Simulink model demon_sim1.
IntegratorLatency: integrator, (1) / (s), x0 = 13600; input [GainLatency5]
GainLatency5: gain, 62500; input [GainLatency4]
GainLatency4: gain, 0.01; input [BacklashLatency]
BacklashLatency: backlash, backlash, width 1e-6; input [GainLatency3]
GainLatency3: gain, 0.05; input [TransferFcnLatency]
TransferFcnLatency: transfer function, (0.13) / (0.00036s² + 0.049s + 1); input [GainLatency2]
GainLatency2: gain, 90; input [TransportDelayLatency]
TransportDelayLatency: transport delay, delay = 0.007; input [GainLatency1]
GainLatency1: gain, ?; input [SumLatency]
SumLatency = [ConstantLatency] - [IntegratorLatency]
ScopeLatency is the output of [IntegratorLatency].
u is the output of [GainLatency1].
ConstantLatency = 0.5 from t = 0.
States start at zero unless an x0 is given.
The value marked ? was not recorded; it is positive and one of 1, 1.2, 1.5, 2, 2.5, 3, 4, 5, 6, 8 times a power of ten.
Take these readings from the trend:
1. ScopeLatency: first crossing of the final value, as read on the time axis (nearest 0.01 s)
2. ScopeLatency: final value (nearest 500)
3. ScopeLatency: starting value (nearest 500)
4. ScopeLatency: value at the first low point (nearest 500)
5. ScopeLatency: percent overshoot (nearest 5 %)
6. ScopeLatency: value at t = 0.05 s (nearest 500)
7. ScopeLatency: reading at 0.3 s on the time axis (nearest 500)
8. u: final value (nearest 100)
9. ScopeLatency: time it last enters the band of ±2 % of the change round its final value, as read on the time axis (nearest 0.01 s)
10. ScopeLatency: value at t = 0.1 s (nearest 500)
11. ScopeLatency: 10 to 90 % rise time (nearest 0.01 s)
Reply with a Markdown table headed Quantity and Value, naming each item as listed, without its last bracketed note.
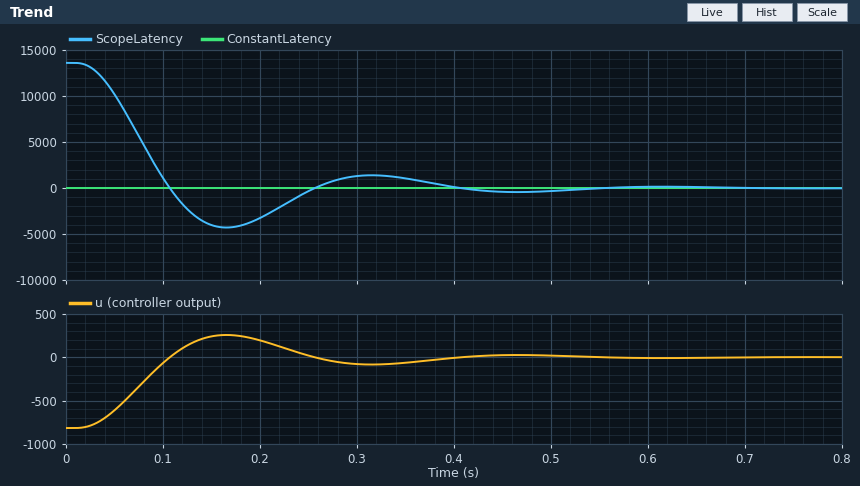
| Quantity | Value |
|---|---|
| ScopeLatency: first crossing of the final value, as read on the time axis | 0.11 s |
| ScopeLatency: final value | 0 |
| ScopeLatency: starting value | 13500 |
| ScopeLatency: value at the first low point | -4500 |
| ScopeLatency: percent overshoot | 30 % |
| ScopeLatency: value at t = 0.05 s | 10000 |
| ScopeLatency: reading at 0.3 s on the time axis | 1500 |
| u: final value | 0 |
| ScopeLatency: time it last enters the band of ±2 % of the change round its final value, as read on the time axis | 0.51 s |
| ScopeLatency: value at t = 0.1 s | 1000 |
| ScopeLatency: 10 to 90 % rise time | 0.06 s |
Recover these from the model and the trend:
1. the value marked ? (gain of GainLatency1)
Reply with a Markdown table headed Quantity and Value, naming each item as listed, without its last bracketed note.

| Quantity | Value |
|---|---|
| the value marked ? | 0.06 |
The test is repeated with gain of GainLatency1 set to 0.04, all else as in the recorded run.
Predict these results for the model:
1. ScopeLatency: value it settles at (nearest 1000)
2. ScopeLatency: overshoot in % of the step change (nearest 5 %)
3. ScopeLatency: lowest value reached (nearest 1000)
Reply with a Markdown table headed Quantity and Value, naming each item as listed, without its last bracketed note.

| Quantity | Value |
|---|---|
| ScopeLatency: value it settles at | 0 |
| ScopeLatency: overshoot in % of the step change | 15 % |
| ScopeLatency: lowest value reached | -2000 |
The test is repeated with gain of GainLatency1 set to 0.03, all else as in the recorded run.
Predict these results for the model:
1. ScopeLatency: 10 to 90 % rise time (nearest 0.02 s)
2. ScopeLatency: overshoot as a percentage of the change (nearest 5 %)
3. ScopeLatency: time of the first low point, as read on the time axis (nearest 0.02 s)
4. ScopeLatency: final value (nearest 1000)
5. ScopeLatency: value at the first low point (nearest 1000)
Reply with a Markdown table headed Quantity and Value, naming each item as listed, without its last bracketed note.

| Quantity | Value |
|---|---|
| ScopeLatency: 10 to 90 % rise time | 0.12 s |
| ScopeLatency: overshoot as a percentage of the change | 10 % |
| ScopeLatency: time of the first low point, as read on the time axis | 0.26 s |
| ScopeLatency: final value | 0 |
| ScopeLatency: value at the first low point | -1000 |
